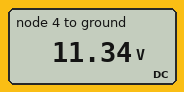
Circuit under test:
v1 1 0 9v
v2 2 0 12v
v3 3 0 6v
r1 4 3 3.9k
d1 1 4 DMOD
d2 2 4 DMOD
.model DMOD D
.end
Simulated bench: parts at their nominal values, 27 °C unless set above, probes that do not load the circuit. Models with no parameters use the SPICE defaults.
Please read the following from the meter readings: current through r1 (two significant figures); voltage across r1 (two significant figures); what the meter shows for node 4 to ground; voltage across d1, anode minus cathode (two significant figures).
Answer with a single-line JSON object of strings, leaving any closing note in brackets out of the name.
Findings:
{"current through r1": "1.4 mA", "voltage across r1": "5.3 V", "what the meter shows for node 4 to ground": "11.34 V", "voltage across d1, anode minus cathode": "-2.3 V"}
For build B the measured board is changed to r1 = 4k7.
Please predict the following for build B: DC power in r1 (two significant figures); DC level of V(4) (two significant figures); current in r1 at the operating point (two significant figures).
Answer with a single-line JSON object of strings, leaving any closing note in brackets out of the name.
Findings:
{"DC power in r1": "6.1 mW", "DC level of V(4)": "11 V", "current in r1 at the operating point": "1.1 mA"}
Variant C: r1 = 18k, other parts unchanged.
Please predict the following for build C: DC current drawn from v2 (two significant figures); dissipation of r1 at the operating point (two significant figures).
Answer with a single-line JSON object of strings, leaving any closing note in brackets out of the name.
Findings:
{"DC current drawn from v2": "300 µA", "dissipation of r1 at the operating point": "1.6 mW"}
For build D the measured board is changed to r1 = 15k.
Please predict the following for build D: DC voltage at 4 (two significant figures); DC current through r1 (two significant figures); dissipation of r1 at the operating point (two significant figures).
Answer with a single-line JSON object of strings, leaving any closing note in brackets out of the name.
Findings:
{"DC voltage at 4": "11 V", "DC current through r1": "360 µA", "dissipation of r1 at the operating point": "1.9 mW"}
